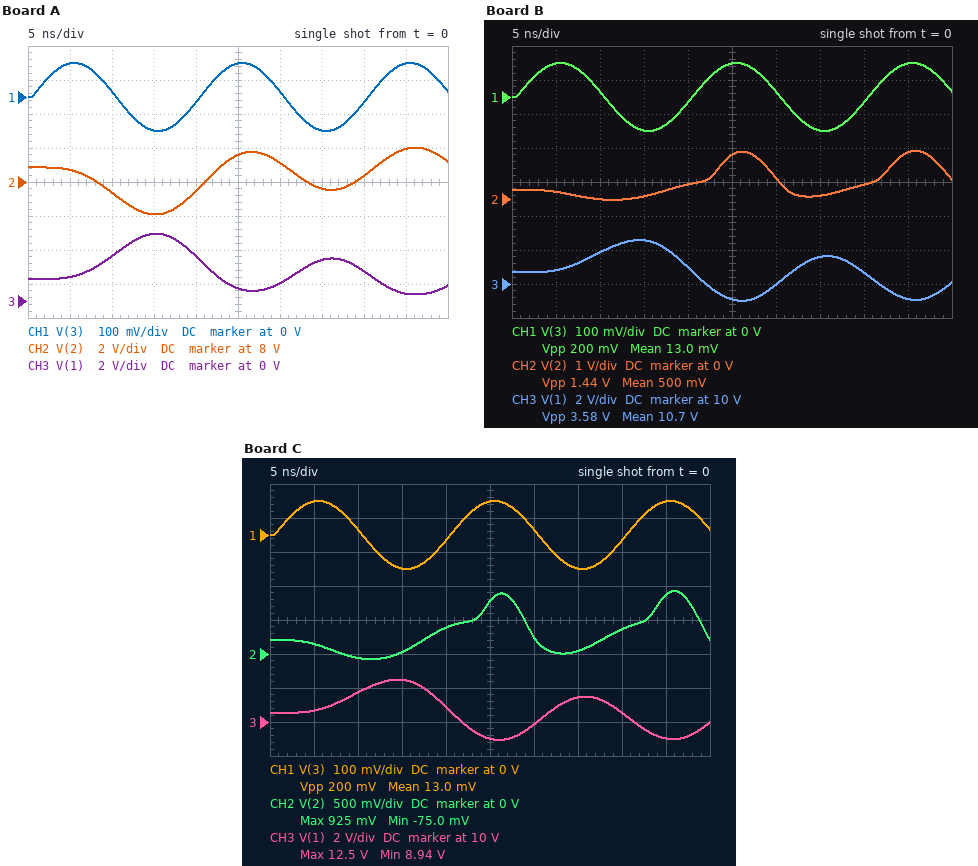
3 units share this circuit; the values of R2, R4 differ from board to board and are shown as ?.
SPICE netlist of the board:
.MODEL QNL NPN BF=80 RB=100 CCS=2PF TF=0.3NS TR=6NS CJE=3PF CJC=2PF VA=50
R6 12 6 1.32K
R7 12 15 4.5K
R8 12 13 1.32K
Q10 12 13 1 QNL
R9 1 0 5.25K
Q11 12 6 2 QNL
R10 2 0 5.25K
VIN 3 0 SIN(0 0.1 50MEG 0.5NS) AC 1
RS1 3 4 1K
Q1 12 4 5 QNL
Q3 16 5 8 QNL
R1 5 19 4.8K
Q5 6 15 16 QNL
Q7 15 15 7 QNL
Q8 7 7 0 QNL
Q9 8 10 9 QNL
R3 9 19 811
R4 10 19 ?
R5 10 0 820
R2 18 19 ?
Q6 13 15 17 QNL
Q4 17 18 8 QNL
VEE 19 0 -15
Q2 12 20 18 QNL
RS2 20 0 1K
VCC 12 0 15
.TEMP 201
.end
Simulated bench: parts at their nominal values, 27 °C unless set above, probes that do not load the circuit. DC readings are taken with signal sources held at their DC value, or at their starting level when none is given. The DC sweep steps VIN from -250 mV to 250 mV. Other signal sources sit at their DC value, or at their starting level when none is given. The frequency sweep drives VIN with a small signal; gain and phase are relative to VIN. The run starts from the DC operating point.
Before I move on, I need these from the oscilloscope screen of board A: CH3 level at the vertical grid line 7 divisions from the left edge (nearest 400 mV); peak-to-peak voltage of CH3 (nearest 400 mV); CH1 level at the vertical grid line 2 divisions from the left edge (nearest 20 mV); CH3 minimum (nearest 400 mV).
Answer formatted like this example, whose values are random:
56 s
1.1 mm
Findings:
2.4 V
3.6 V
20 mV
400 mV
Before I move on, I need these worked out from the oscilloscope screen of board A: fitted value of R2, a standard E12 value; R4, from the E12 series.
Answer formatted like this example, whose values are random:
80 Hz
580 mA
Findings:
10 kΩ
4.7 kΩ
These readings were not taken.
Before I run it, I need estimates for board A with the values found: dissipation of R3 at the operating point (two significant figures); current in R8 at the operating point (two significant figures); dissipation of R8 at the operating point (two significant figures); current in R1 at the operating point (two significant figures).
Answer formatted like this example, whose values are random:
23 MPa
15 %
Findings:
180 mW
10 mA
130 mW
3.0 mA
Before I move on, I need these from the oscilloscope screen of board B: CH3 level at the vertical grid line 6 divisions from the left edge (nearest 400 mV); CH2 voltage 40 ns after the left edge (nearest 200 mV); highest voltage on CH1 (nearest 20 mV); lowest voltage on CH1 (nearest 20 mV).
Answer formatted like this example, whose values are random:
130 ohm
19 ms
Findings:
10.0 V
400 mV
100 mV
-100 mV
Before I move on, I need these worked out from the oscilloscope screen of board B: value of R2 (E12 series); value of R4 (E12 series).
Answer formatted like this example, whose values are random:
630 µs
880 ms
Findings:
2.2 kΩ
3.9 kΩ
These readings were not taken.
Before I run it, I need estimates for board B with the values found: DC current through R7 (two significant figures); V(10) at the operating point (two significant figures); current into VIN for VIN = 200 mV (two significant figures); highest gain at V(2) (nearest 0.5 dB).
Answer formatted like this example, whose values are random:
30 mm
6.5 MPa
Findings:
3.1 mA
-2.7 V
-31 µA
22.5 dB
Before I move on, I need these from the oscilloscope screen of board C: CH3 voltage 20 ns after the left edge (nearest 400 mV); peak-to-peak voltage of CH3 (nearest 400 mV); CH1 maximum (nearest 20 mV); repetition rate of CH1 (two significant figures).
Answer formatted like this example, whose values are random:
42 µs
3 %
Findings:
10.8 V
3.6 V
100 mV
50 MHz
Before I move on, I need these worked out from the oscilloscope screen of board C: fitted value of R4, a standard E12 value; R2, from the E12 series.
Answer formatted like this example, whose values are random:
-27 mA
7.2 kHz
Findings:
4.7 kΩ
2.2 kΩ
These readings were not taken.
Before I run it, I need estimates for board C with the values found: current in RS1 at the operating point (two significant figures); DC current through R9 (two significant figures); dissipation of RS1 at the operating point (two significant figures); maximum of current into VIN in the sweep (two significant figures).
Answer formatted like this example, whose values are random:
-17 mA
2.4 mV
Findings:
30 µA
2.0 mA
890 nW
-28 µA
